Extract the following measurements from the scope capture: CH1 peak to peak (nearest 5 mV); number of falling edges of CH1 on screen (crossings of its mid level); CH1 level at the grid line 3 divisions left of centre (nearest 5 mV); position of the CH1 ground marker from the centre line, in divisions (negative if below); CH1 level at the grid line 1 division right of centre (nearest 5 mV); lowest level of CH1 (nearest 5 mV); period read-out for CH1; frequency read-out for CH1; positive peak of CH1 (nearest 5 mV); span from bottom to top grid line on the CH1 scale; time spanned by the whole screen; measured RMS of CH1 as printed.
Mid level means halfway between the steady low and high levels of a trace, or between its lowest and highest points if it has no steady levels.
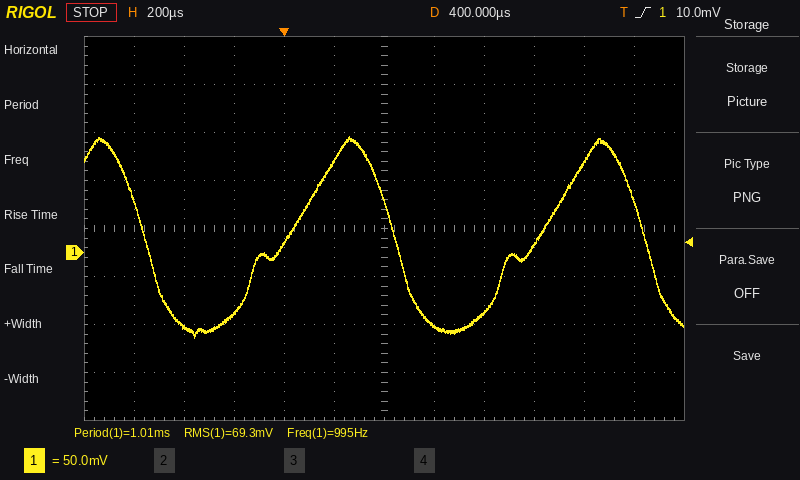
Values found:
210 mV
3
-65 mV
-0.5 div
-75 mV
-90 mV
1.01 ms
995 Hz
120 mV
400 mV
2.4 ms
69.3 mV
